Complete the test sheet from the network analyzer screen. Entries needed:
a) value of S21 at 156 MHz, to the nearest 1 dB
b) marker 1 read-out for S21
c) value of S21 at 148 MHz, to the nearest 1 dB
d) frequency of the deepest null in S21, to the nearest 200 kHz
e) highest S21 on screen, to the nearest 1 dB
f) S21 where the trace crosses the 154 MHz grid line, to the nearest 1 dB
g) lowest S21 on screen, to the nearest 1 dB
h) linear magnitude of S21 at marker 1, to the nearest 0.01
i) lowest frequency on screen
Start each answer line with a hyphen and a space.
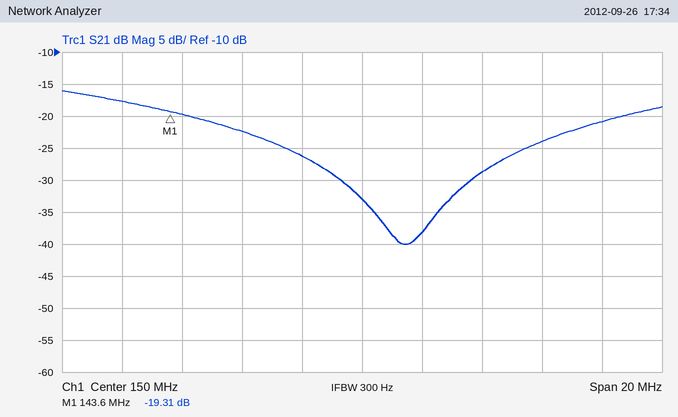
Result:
- -24 dB
- -19.31 dB
- -26 dB
- 151.4 MHz
- -16 dB
- -29 dB
- -40 dB
- 0.11
- 140 MHz
